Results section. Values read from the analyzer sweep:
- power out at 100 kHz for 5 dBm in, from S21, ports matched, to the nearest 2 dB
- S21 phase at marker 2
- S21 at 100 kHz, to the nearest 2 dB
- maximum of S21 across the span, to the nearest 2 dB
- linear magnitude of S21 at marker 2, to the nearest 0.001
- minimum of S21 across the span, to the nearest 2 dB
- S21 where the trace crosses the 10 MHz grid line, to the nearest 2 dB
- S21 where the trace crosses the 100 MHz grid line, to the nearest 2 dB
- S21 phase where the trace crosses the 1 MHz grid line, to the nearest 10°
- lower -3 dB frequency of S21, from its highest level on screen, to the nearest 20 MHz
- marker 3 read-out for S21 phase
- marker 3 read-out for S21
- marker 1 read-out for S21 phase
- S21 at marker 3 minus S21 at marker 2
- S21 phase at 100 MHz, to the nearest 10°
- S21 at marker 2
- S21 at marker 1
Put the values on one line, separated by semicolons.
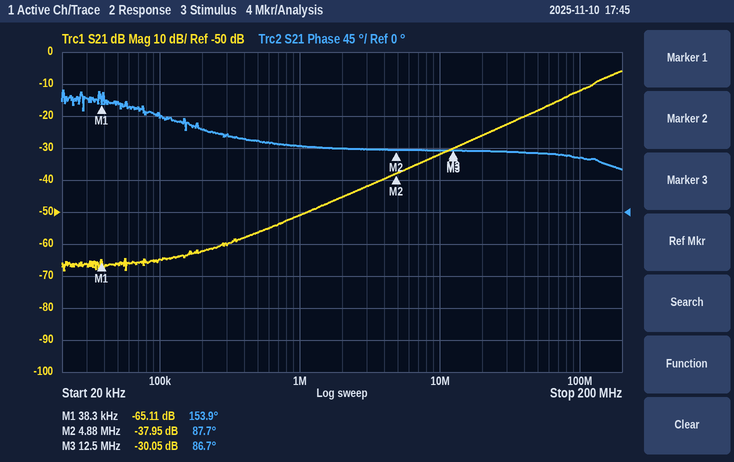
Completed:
-60 dBm; 87.7°; -64 dB; -6 dB; 0.013; -68 dB; -32 dB; -12 dB; 90°; 140 MHz; 86.7°; -30.05 dB; 153.9°; 7.90 dB; 80°; -37.95 dB; -65.11 dB
